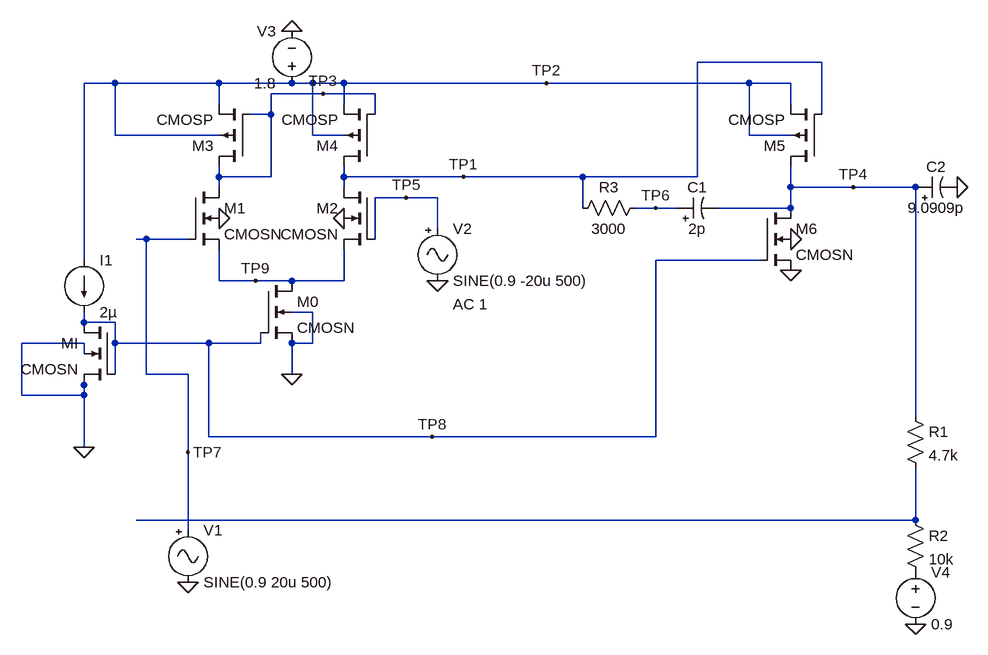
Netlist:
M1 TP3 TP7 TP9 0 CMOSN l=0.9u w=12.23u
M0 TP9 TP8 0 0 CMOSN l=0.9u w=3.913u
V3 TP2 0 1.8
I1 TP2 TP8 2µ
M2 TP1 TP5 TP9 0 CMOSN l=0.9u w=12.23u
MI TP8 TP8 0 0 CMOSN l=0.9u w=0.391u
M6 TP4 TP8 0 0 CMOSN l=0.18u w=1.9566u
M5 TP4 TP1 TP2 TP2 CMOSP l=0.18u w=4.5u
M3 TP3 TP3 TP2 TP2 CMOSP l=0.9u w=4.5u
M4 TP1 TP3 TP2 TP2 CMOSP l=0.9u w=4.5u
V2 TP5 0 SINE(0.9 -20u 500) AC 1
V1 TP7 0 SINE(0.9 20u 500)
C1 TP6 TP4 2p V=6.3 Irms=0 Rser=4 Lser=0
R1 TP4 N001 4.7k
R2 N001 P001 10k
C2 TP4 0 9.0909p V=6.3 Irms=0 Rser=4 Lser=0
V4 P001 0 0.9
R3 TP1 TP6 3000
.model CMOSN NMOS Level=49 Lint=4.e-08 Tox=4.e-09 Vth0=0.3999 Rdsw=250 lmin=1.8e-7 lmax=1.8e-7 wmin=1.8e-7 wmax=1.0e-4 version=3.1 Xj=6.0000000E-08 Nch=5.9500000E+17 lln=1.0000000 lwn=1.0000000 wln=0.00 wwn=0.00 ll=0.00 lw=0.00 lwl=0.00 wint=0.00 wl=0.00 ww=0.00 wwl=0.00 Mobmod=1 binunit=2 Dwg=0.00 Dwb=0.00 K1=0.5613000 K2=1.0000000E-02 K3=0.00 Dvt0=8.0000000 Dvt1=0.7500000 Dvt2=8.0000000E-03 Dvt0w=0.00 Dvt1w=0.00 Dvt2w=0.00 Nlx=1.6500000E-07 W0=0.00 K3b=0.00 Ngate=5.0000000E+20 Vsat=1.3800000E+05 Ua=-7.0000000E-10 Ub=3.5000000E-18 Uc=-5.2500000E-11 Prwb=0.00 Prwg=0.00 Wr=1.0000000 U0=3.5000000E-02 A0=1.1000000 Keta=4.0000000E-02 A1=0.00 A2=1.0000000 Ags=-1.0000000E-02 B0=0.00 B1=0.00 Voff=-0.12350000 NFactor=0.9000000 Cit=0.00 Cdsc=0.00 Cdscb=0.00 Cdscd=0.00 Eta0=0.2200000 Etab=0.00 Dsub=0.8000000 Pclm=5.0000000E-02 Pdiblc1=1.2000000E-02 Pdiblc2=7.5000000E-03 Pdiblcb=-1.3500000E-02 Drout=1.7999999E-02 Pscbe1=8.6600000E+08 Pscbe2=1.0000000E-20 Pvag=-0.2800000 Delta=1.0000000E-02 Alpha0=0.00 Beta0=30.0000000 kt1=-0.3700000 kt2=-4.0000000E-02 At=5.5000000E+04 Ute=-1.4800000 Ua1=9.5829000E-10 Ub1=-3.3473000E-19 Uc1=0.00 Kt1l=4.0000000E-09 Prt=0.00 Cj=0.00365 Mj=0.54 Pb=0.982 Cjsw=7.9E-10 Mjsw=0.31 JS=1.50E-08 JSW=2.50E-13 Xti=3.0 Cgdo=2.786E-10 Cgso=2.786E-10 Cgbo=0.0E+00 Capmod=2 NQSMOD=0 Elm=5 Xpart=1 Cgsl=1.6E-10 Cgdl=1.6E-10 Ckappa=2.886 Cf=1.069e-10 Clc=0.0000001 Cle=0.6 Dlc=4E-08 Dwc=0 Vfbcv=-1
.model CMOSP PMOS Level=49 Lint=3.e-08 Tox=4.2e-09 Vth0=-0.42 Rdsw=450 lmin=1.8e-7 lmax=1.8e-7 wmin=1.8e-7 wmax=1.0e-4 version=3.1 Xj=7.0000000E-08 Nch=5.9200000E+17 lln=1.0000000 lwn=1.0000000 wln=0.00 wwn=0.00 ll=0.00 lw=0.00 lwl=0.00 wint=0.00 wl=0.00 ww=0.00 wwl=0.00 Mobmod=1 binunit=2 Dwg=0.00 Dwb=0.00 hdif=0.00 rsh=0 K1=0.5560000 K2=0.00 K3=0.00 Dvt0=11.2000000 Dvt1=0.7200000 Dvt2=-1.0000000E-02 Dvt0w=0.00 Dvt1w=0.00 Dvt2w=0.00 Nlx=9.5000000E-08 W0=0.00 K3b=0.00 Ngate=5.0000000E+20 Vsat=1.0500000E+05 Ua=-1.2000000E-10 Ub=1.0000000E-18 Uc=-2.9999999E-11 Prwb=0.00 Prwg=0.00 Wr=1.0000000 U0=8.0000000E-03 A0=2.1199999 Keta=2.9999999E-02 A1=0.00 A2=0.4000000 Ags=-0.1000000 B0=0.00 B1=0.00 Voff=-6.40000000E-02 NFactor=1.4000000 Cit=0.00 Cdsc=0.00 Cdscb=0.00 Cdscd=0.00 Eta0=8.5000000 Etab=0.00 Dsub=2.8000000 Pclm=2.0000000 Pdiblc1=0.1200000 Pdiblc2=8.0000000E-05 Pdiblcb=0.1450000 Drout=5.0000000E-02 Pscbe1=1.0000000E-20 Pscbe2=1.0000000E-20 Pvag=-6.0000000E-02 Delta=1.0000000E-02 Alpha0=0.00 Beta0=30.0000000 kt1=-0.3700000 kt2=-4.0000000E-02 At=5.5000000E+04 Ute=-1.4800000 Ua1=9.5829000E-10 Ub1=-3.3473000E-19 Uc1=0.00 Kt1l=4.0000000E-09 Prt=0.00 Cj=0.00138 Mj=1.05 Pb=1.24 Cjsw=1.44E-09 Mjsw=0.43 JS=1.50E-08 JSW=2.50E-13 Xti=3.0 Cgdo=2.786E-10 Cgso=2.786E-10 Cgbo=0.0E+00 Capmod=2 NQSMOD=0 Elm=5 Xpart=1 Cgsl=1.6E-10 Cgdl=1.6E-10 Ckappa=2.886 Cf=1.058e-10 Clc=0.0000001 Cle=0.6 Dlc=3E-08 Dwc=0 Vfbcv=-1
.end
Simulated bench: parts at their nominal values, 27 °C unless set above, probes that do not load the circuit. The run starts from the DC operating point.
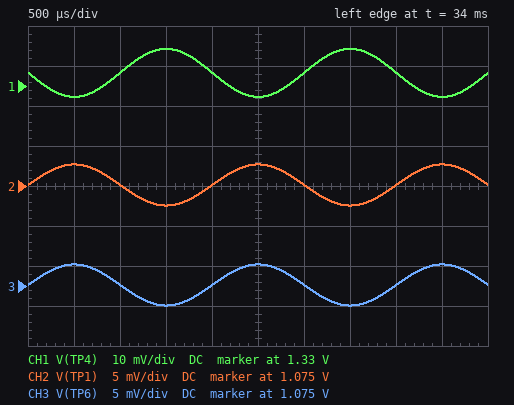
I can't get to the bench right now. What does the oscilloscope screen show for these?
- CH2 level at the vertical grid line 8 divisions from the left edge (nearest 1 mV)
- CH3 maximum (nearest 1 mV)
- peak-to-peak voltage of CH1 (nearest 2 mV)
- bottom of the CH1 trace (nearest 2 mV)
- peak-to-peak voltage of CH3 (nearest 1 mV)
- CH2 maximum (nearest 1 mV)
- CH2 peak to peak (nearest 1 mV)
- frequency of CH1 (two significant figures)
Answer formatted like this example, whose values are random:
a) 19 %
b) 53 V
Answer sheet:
a) 1.075 V
b) 1.078 V
c) 12 mV
d) 1.328 V
e) 5 mV
f) 1.078 V
g) 5 mV
h) 500 Hz
